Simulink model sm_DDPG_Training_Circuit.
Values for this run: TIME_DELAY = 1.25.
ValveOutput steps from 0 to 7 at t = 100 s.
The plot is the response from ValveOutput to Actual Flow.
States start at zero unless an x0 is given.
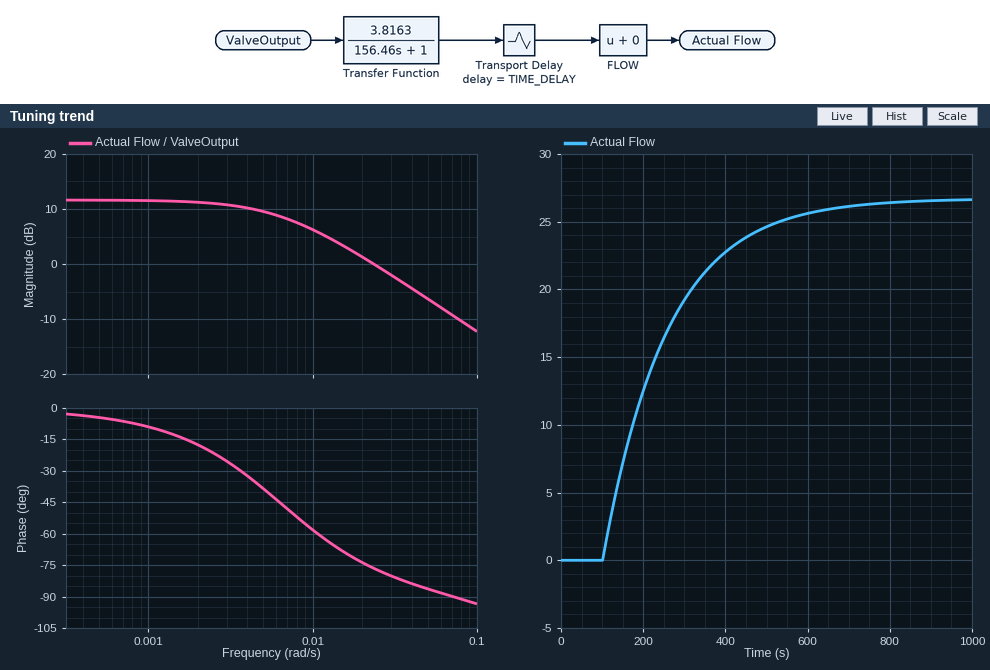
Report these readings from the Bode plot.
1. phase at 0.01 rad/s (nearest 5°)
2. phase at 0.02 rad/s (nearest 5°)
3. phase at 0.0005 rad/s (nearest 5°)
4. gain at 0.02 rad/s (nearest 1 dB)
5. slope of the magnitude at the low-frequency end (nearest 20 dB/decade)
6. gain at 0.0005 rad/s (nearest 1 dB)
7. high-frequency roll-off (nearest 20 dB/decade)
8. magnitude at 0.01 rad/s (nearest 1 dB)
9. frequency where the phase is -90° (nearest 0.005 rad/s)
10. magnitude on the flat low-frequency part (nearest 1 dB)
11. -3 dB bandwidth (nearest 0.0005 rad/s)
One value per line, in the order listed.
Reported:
-60°
-75°
-5°
1 dB
0 dB/decade
12 dB
-20 dB/decade
6 dB
0.070 rad/s
12 dB
0.0065 rad/s
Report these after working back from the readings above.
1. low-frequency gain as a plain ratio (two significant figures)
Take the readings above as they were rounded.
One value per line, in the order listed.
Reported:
4.0
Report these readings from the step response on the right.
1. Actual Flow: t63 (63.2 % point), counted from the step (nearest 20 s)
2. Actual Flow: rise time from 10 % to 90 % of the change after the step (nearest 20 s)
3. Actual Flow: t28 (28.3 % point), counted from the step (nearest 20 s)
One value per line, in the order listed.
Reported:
160 s
340 s
60 s
